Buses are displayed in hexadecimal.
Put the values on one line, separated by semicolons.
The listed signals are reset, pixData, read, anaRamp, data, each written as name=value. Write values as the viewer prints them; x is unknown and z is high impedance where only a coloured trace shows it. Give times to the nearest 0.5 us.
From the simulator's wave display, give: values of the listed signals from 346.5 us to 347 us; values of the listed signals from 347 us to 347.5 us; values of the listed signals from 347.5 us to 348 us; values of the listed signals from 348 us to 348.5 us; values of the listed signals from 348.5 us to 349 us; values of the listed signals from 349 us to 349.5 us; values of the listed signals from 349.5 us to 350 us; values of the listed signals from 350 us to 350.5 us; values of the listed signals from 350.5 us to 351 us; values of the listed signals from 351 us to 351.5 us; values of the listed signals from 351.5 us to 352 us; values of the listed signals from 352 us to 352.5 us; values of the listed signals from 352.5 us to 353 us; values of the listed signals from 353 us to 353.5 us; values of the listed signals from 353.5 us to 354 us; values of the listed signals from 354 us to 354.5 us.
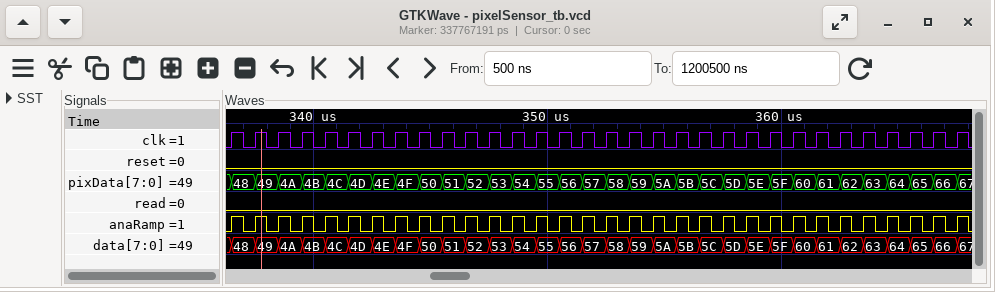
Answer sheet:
reset=0, pixData=52, read=0, anaRamp=1, data=52; reset=0, pixData=52, read=0, anaRamp=0, data=52; reset=0, pixData=53, read=0, anaRamp=1, data=53; reset=0, pixData=53, read=0, anaRamp=0, data=53; reset=0, pixData=54, read=0, anaRamp=1, data=54; reset=0, pixData=54, read=0, anaRamp=0, data=54; reset=0, pixData=55, read=0, anaRamp=1, data=55; reset=0, pixData=55, read=0, anaRamp=0, data=55; reset=0, pixData=56, read=0, anaRamp=1, data=56; reset=0, pixData=56, read=0, anaRamp=0, data=56; reset=0, pixData=57, read=0, anaRamp=1, data=57; reset=0, pixData=57, read=0, anaRamp=0, data=57; reset=0, pixData=58, read=0, anaRamp=1, data=58; reset=0, pixData=58, read=0, anaRamp=0, data=58; reset=0, pixData=59, read=0, anaRamp=1, data=59; reset=0, pixData=59, read=0, anaRamp=0, data=59
